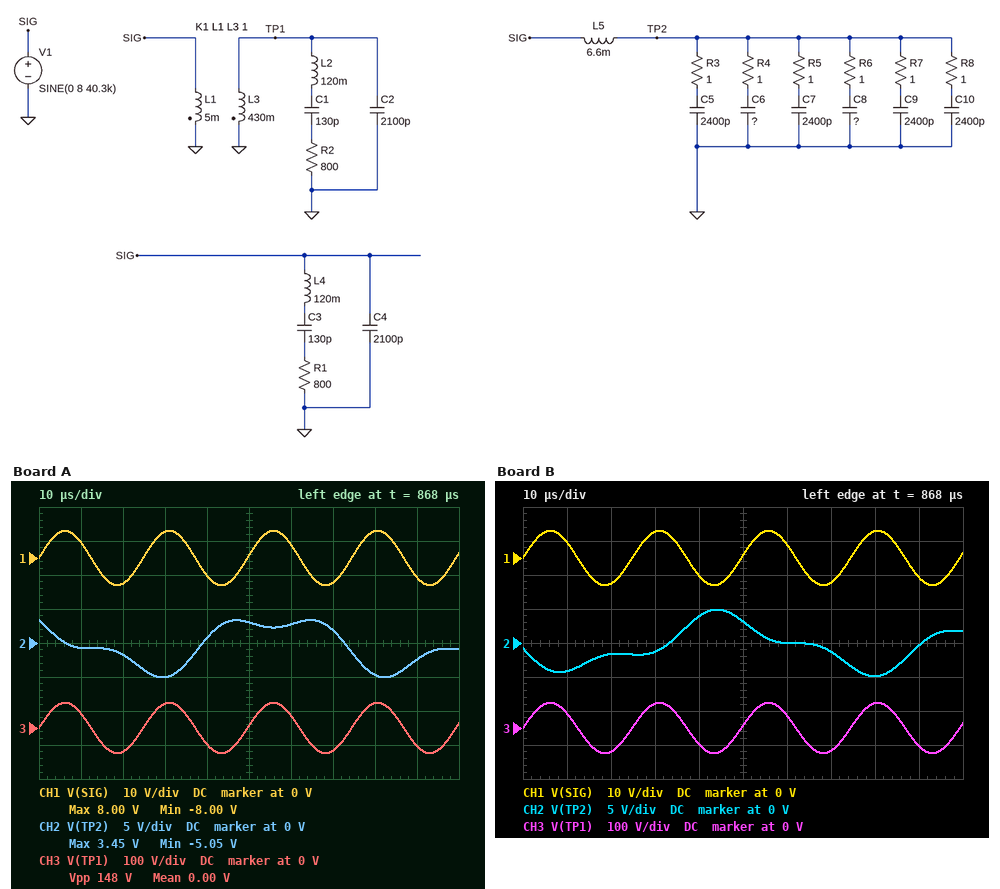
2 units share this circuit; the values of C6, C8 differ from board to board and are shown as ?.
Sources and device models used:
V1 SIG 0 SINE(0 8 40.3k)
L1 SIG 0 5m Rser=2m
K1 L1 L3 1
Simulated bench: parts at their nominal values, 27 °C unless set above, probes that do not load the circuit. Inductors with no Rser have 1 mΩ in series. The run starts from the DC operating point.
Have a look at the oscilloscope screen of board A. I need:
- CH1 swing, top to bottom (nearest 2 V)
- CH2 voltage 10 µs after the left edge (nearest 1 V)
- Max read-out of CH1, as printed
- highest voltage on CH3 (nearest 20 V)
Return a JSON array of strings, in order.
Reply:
["16 V", "-1 V", "8.00 V", "80 V"]
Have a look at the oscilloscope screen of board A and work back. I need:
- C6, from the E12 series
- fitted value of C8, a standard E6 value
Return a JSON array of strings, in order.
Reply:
["1.2 nF", "3.3 nF"]
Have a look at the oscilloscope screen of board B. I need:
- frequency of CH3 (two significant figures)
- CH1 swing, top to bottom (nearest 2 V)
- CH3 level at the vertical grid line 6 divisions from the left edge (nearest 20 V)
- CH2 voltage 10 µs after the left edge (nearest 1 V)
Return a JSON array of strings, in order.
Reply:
["40 kHz", "16 V", "40 V", "-4 V"]
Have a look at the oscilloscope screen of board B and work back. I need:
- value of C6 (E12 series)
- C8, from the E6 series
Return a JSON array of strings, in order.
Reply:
["1.5 nF", "4.7 nF"]
